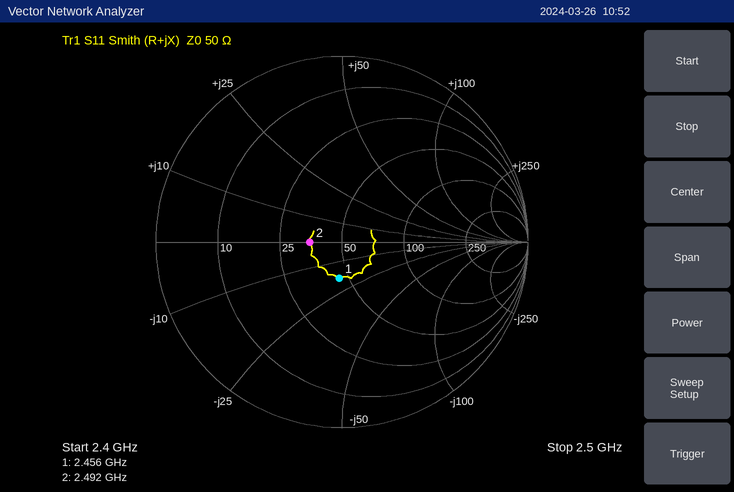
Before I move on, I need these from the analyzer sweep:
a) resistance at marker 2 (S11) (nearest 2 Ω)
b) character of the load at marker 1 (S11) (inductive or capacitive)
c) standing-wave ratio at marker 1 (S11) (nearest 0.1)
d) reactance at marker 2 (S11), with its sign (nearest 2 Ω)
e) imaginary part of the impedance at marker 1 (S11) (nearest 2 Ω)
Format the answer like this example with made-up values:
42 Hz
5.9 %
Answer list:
36 Ω
capacitive
1.5
0 Ω
-18 Ω
